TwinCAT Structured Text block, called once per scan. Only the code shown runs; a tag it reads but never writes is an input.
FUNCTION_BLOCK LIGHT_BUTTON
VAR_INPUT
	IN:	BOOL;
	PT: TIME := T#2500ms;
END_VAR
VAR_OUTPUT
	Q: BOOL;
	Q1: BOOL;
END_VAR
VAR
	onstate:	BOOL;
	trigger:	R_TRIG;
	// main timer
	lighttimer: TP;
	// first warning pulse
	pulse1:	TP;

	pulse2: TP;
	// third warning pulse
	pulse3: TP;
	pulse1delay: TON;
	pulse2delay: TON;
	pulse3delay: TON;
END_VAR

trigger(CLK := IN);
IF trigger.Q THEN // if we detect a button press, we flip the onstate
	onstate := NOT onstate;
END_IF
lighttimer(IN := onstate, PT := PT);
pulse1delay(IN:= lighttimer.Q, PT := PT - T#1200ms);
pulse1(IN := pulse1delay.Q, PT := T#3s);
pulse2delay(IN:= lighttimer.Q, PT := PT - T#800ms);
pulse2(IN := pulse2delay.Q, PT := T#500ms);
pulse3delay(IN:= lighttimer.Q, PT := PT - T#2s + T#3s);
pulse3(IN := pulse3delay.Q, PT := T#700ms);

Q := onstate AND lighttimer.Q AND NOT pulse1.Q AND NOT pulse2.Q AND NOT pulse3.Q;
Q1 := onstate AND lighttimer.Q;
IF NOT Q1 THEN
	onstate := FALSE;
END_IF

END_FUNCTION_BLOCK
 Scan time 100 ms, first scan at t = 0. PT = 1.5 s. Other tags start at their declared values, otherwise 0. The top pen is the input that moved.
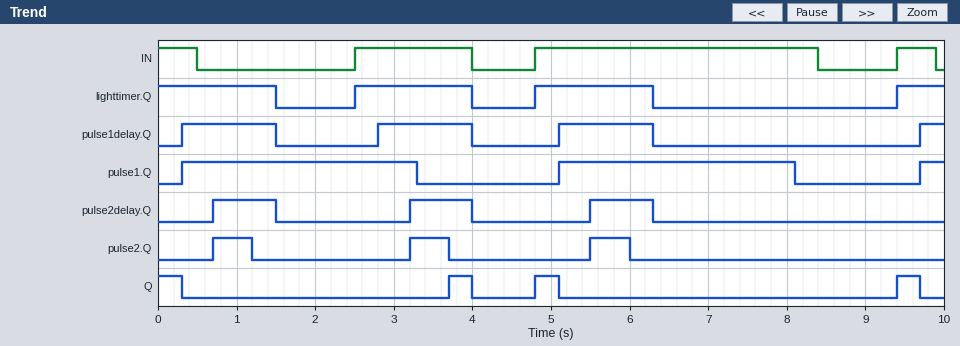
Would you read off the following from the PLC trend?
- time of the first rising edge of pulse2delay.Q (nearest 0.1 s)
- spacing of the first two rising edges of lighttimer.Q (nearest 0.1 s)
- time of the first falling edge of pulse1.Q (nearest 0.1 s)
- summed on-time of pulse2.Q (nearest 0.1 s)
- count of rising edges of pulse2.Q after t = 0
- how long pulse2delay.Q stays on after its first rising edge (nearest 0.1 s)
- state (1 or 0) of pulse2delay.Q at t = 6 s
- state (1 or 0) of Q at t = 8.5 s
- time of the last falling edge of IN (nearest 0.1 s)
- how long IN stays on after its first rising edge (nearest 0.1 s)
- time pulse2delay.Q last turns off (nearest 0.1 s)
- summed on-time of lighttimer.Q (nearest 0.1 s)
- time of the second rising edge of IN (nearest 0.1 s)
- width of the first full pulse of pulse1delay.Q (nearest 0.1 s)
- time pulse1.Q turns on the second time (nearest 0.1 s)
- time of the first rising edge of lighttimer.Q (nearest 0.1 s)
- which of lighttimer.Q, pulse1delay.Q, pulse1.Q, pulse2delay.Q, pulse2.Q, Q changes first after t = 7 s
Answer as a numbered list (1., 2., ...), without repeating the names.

1. 0.7 s
2. 2.3 s
3. 3.3 s
4. 1.5 s
5. 3
6. 0.8 s
7. 1
8. 0
9. 9.9 s
10. 1.5 s
11. 6.3 s
12. 5.1 s
13. 4.8 s
14. 1.2 s
15. 5.1 s
16. 2.5 s
17. pulse1.Q
